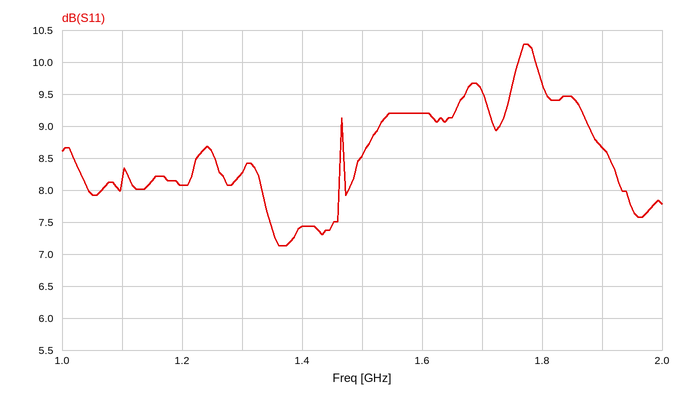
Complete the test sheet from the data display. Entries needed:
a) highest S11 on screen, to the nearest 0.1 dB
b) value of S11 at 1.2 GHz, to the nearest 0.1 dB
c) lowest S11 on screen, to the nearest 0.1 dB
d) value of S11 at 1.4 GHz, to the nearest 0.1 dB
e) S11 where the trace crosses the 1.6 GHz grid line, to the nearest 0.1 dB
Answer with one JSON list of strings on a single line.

["10.3 dB", "8.1 dB", "7.1 dB", "7.4 dB", "9.2 dB"]
